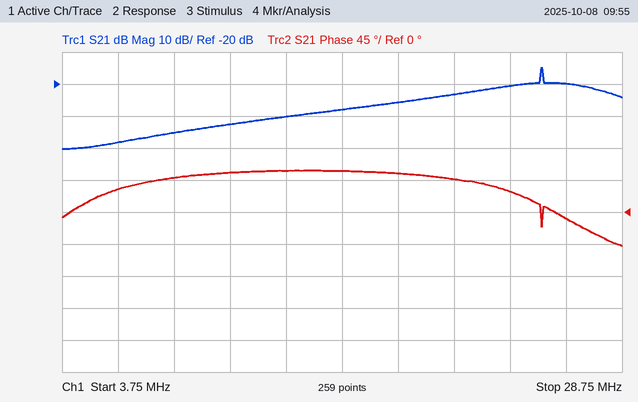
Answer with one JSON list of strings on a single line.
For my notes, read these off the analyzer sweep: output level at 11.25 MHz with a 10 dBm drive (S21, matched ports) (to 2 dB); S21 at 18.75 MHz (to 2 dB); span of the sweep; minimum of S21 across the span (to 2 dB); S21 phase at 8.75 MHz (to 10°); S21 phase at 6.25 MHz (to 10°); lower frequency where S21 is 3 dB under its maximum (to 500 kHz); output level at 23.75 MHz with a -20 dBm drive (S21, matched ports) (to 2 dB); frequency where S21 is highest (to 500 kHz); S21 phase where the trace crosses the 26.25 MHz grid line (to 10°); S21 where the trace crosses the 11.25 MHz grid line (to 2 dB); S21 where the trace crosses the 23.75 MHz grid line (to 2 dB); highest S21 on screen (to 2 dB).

["-22 dBm", "-26 dB", "25 MHz", "-40 dB", "50°", "30°", "25.0 MHz", "-40 dBm", "25.0 MHz", "-10°", "-32 dB", "-20 dB", "-14 dB"]
